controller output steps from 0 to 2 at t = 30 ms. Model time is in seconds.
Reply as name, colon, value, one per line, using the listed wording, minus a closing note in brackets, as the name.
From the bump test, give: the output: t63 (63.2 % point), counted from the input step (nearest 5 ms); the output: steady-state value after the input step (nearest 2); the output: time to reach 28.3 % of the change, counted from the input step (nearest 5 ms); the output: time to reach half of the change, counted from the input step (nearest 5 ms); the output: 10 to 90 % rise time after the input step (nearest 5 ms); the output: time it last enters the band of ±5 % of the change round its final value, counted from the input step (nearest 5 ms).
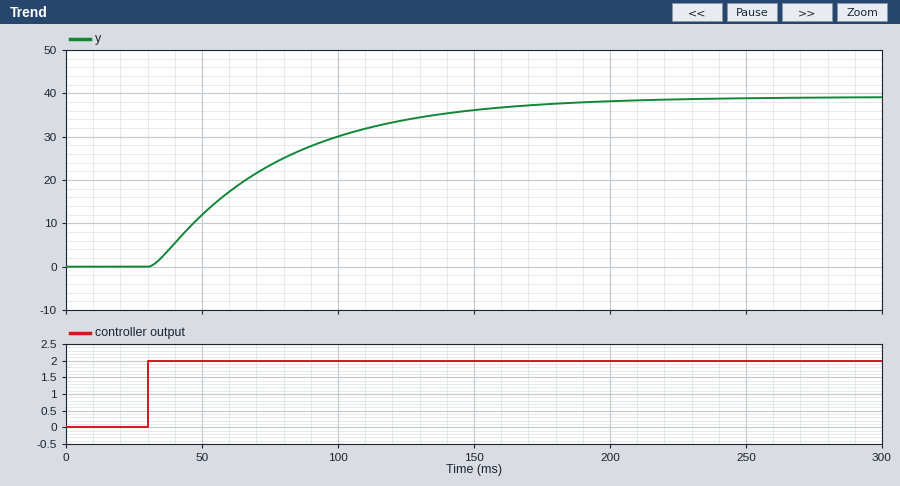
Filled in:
the output: t63 (63.2 % point), counted from the input step: 50 ms
the output: steady-state value after the input step: 40
the output: time to reach 28.3 % of the change, counted from the input step: 20 ms
the output: time to reach half of the change, counted from the input step: 35 ms
the output: 10 to 90 % rise time after the input step: 100 ms
the output: time it last enters the band of ±5 % of the change round its final value, counted from the input step: 140 ms
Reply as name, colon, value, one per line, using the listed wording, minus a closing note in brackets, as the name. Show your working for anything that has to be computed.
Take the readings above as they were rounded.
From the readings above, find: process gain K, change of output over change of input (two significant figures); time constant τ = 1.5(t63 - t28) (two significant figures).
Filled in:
process gain K, change of output over change of input: (40 - 0) / 2 = 20
time constant τ = 1.5(t63 - t28): 1.5 × (50 - 20) = 45 ms
